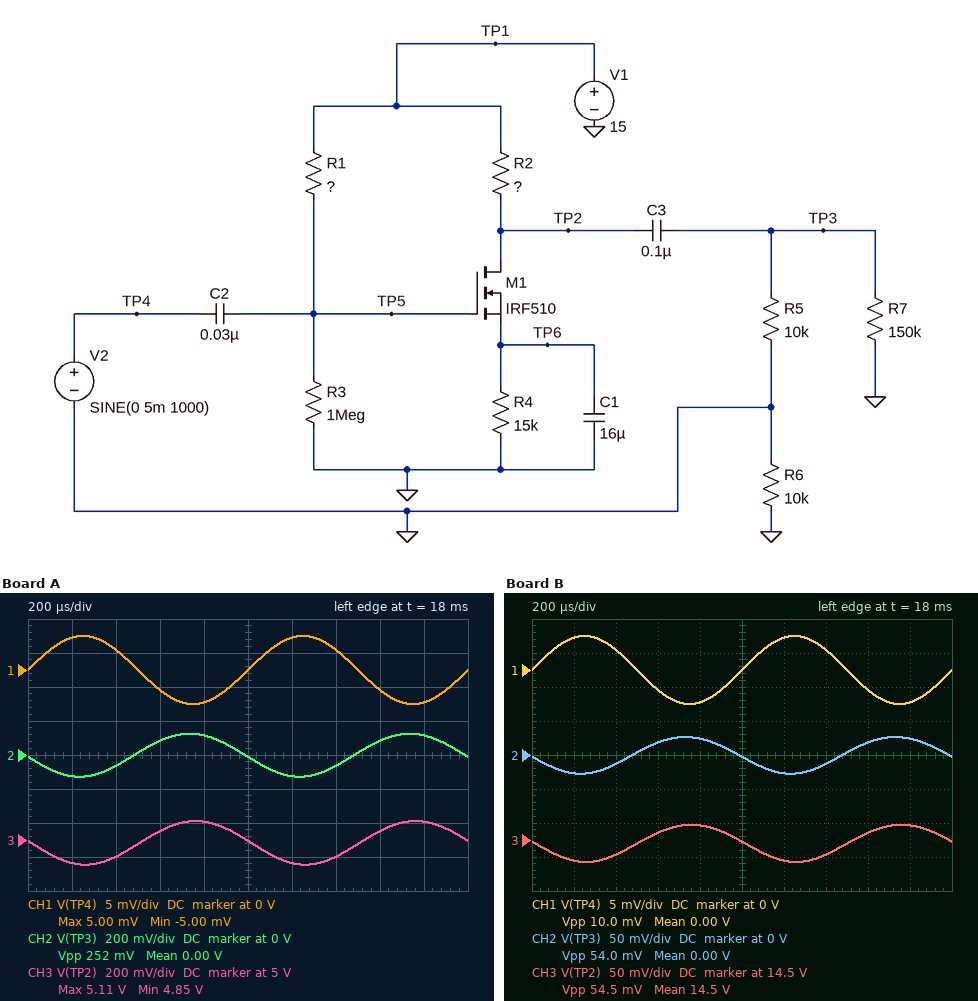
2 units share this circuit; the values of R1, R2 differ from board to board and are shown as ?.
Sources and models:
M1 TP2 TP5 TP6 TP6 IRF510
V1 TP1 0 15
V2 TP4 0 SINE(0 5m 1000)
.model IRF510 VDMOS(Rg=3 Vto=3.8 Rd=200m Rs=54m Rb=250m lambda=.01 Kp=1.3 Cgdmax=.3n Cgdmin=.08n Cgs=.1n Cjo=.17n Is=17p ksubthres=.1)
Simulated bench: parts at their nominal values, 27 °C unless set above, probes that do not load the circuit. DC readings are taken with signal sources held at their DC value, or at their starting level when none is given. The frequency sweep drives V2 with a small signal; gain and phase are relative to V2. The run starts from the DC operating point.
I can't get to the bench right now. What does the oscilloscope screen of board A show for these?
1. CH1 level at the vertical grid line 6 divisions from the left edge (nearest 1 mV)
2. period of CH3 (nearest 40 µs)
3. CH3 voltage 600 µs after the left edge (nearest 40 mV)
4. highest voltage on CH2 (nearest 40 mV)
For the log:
5 mV
1.00 ms
5.04 V
120 mV
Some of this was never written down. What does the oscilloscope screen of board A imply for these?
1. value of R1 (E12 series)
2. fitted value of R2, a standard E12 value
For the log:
1 MΩ
39 kΩ
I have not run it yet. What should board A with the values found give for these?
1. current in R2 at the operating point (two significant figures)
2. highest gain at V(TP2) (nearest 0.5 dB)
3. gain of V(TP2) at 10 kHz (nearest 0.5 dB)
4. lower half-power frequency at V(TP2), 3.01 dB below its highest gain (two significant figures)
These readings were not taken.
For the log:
260 µA
32.5 dB
28.0 dB
12 Hz
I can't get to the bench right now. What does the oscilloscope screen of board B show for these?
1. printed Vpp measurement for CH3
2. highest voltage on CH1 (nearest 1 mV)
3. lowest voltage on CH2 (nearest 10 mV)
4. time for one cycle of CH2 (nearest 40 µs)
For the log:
54.5 mV
5 mV
-30 mV
1.00 ms
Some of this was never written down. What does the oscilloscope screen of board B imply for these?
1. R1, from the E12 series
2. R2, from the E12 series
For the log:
2.2 MΩ
6.8 kΩ
